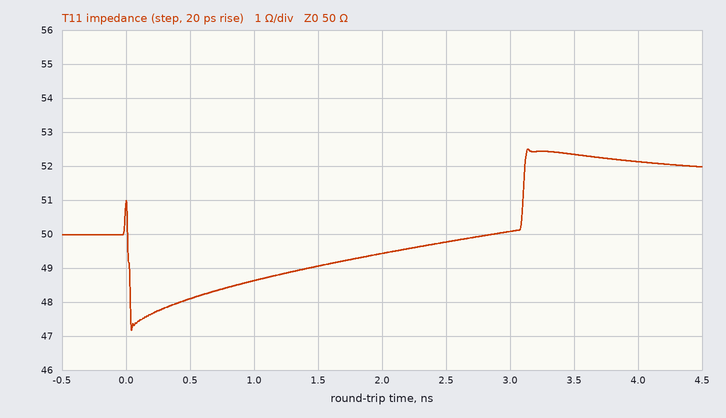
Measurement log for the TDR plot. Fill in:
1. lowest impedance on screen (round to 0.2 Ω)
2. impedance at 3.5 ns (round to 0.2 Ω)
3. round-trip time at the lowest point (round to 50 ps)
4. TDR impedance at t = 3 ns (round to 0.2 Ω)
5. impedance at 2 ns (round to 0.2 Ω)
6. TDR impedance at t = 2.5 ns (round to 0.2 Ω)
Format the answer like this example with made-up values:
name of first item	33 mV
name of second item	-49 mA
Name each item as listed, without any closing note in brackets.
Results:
lowest impedance on screen	47.2 Ω
impedance at 3.5 ns	52.4 Ω
round-trip time at the lowest point	50 ps
TDR impedance at t = 3 ns	50.0 Ω
impedance at 2 ns	49.4 Ω
TDR impedance at t = 2.5 ns	49.8 Ω
